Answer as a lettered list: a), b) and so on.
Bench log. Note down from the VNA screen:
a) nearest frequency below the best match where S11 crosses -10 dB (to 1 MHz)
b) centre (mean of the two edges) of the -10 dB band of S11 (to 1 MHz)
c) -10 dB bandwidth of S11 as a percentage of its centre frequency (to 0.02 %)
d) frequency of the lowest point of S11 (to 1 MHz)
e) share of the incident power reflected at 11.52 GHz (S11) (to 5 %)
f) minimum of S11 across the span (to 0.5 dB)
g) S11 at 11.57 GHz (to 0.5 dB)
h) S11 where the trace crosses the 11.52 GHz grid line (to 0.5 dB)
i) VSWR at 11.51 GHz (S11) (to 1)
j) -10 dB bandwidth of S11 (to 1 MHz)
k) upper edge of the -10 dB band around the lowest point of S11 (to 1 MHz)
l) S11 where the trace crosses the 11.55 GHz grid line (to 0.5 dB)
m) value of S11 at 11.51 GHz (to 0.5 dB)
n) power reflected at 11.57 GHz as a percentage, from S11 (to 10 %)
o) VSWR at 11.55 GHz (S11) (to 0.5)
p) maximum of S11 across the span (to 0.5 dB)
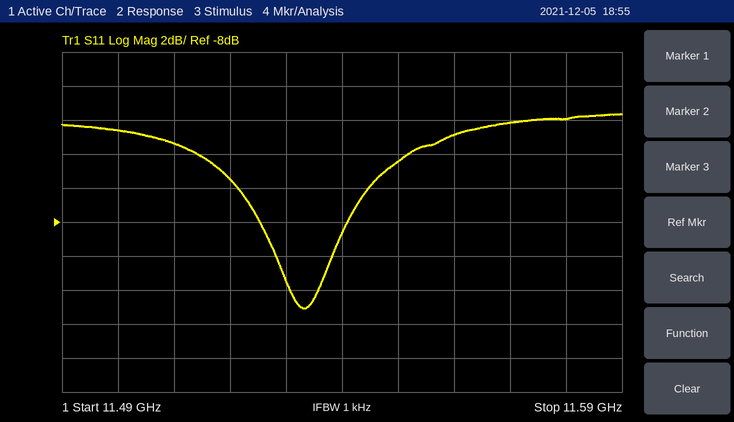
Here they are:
a) 11.528 GHz
b) 11.533 GHz
c) 0.08 %
d) 11.533 GHz
e) 30 %
f) -13.0 dB
g) -2.0 dB
h) -5.5 dB
i) 5
j) 10 MHz
k) 11.538 GHz
l) -4.5 dB
m) -3.5 dB
n) 60 %
o) 4.0
p) -1.5 dB
